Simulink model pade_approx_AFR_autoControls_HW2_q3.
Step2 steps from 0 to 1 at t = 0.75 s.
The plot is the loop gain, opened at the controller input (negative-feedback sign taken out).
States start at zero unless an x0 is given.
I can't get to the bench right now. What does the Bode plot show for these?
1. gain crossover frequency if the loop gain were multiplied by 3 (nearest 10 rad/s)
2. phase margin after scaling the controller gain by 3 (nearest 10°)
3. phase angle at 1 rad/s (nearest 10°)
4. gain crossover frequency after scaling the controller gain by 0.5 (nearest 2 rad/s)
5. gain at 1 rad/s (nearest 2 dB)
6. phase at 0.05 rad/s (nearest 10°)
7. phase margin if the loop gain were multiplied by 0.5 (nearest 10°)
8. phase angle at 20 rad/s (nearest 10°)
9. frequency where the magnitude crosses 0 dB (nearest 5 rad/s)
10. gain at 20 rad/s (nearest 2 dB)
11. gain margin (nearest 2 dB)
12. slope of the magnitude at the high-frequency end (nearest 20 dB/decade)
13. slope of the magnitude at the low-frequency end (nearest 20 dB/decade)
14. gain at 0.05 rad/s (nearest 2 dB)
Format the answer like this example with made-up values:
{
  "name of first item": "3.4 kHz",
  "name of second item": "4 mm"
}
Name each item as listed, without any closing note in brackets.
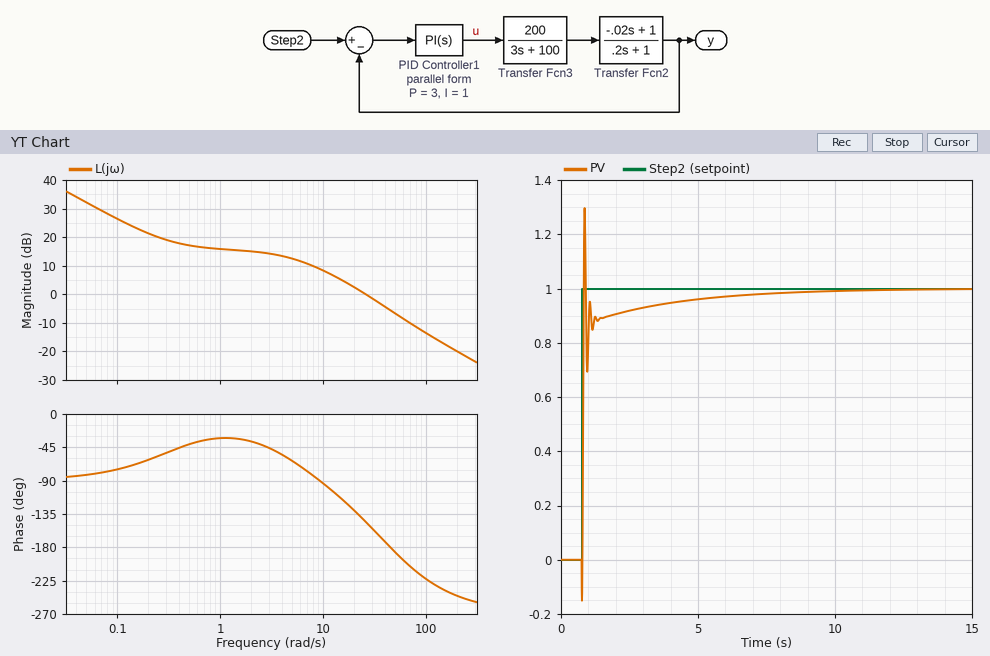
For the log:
{
  "gain crossover frequency if the loop gain were multiplied by 3": "70 rad/s",
  "phase margin after scaling the controller gain by 3": "-20°",
  "phase angle at 1 rad/s": "-30°",
  "gain crossover frequency after scaling the controller gain by 0.5": "14 rad/s",
  "gain at 1 rad/s": "16 dB",
  "phase at 0.05 rad/s": "-80°",
  "phase margin if the loop gain were multiplied by 0.5": "70°",
  "phase angle at 20 rad/s": "-130°",
  "frequency where the magnitude crosses 0 dB": "25 rad/s",
  "gain at 20 rad/s": "2 dB",
  "gain margin": "6 dB",
  "slope of the magnitude at the high-frequency end": "-20 dB/decade",
  "slope of the magnitude at the low-frequency end": "-20 dB/decade",
  "gain at 0.05 rad/s": "32 dB"
}
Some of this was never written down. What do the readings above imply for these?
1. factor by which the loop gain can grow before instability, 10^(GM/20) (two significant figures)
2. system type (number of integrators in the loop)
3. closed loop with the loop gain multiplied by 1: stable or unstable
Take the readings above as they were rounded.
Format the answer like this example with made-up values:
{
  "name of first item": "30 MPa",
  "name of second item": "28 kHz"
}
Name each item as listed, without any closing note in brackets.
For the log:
{
  "factor by which the loop gain can grow before instability, 10^(GM/20)": "2.0",
  "system type": "1",
  "closed loop with the loop gain multiplied by 1: stable or unstable": "stable"
}
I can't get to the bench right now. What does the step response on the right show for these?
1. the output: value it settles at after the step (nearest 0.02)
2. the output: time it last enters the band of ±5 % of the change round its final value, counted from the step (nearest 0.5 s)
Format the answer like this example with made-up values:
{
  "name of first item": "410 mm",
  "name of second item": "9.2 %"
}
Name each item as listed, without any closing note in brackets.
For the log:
{
  "the output: value it settles at after the step": "1.00",
  "the output: time it last enters the band of ±5 % of the change round its final value, counted from the step": "3.5 s"
}
